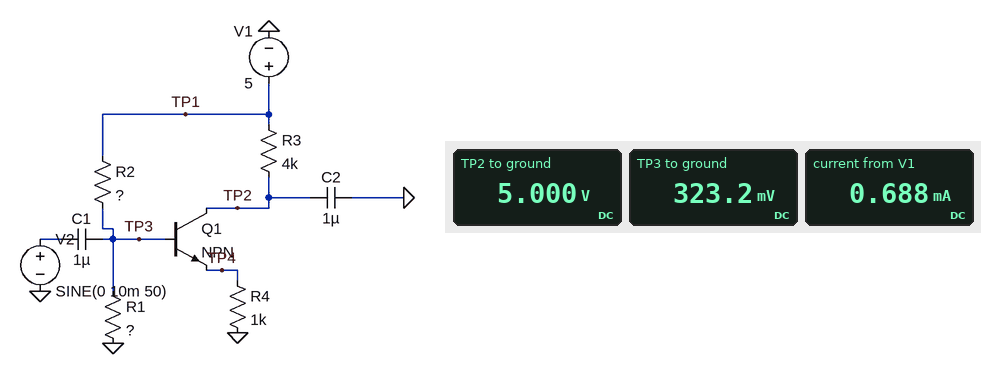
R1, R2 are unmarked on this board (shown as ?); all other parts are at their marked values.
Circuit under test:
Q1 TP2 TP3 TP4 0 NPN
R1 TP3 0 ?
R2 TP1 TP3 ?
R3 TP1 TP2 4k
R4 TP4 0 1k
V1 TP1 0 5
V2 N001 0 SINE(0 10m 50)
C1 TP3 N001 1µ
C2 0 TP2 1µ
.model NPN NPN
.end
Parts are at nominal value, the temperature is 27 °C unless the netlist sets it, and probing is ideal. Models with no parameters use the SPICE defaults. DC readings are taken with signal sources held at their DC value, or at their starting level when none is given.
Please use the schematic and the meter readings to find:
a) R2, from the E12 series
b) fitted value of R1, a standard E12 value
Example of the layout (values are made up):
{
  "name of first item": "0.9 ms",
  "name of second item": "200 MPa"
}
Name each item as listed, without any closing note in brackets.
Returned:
{
  "R2, from the E12 series": "6.8 kΩ",
  "fitted value of R1, a standard E12 value": "470 Ω"
}
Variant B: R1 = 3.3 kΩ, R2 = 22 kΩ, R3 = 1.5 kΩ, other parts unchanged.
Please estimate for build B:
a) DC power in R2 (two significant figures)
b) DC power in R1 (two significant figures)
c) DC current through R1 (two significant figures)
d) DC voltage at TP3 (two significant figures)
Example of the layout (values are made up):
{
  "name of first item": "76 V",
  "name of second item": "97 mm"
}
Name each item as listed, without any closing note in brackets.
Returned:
{
  "DC power in R2": "860 µW",
  "DC power in R1": "130 µW",
  "DC current through R1": "200 µA",
  "DC voltage at TP3": "650 mV"
}
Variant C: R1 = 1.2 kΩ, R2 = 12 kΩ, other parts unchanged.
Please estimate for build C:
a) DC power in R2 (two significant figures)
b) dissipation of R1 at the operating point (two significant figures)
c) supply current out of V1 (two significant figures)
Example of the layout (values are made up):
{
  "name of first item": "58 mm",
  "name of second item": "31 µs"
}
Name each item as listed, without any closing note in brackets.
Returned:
{
  "DC power in R2": "1.7 mW",
  "dissipation of R1 at the operating point": "170 µW",
  "supply current out of V1": "380 µA"
}
